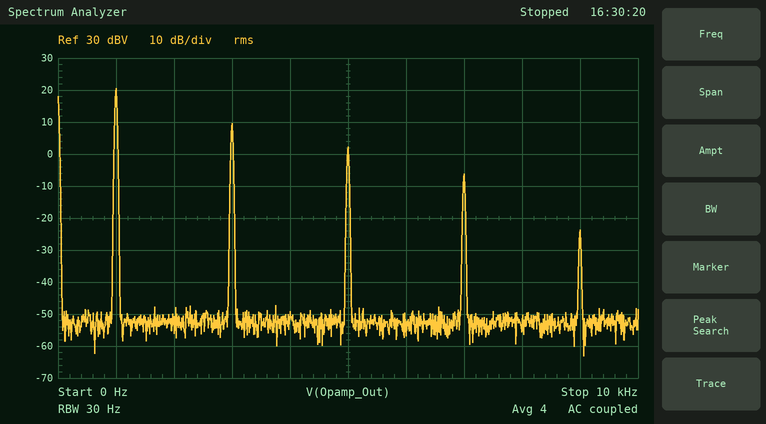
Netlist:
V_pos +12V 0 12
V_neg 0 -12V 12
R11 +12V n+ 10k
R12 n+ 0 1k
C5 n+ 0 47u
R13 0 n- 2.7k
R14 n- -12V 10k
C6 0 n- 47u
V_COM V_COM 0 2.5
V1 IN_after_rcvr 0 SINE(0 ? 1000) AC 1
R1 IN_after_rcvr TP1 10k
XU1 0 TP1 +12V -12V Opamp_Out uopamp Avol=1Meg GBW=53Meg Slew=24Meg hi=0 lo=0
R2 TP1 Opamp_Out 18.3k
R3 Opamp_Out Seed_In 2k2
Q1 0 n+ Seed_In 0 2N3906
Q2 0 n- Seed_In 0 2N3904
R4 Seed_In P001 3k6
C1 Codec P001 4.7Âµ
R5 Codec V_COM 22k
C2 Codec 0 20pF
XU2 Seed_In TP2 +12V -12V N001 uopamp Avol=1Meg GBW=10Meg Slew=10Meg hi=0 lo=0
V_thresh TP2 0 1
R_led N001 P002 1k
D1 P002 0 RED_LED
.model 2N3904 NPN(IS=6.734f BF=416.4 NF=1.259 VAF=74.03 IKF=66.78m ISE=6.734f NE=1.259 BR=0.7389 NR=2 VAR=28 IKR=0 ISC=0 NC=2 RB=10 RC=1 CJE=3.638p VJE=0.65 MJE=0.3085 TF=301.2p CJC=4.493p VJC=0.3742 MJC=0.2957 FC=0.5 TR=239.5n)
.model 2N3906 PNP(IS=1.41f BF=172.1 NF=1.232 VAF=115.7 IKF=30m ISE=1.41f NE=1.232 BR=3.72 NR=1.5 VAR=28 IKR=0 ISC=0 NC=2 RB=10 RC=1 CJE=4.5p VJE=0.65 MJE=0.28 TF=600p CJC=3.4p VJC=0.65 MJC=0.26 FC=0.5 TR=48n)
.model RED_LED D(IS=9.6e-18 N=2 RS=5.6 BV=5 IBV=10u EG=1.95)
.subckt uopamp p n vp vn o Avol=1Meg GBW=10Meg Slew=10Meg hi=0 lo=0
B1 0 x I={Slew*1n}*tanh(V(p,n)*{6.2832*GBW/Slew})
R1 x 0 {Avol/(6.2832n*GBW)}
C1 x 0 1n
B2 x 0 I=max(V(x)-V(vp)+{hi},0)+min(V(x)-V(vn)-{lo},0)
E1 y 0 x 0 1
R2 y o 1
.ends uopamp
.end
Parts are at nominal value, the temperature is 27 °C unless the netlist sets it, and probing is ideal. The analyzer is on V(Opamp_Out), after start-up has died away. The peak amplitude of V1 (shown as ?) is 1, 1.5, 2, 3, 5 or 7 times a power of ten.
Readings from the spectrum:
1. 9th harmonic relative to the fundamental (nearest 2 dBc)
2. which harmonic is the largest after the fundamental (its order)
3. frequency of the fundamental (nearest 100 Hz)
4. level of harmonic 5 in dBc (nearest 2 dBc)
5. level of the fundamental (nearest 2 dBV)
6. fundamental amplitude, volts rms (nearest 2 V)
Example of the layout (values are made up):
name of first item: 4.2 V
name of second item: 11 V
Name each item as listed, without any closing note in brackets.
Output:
9th harmonic relative to the fundamental: -44 dBc
which harmonic is the largest after the fundamental: 3
frequency of the fundamental: 1.0 kHz
level of harmonic 5 in dBc: -18 dBc
level of the fundamental: 20 dBV
fundamental amplitude, volts rms: 10 V
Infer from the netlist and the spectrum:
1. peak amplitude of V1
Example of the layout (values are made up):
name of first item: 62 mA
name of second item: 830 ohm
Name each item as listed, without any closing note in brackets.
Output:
peak amplitude of V1: 20 V
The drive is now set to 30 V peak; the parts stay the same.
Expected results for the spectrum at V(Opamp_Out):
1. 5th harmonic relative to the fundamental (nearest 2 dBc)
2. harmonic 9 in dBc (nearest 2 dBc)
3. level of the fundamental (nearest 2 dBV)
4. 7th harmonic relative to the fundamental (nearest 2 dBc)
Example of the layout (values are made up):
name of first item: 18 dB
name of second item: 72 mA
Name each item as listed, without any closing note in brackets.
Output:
5th harmonic relative to the fundamental: -16 dBc
harmonic 9 in dBc: -26 dBc
level of the fundamental: 20 dBV
7th harmonic relative to the fundamental: -20 dBc
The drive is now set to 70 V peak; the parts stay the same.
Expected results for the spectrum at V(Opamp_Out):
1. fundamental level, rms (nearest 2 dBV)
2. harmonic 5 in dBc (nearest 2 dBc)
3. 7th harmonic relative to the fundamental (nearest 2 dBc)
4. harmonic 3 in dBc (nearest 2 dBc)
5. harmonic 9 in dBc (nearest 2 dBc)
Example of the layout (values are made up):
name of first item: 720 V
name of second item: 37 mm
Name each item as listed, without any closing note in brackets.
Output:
fundamental level, rms: 20 dBV
harmonic 5 in dBc: -14 dBc
7th harmonic relative to the fundamental: -18 dBc
harmonic 3 in dBc: -10 dBc
harmonic 9 in dBc: -20 dBc
